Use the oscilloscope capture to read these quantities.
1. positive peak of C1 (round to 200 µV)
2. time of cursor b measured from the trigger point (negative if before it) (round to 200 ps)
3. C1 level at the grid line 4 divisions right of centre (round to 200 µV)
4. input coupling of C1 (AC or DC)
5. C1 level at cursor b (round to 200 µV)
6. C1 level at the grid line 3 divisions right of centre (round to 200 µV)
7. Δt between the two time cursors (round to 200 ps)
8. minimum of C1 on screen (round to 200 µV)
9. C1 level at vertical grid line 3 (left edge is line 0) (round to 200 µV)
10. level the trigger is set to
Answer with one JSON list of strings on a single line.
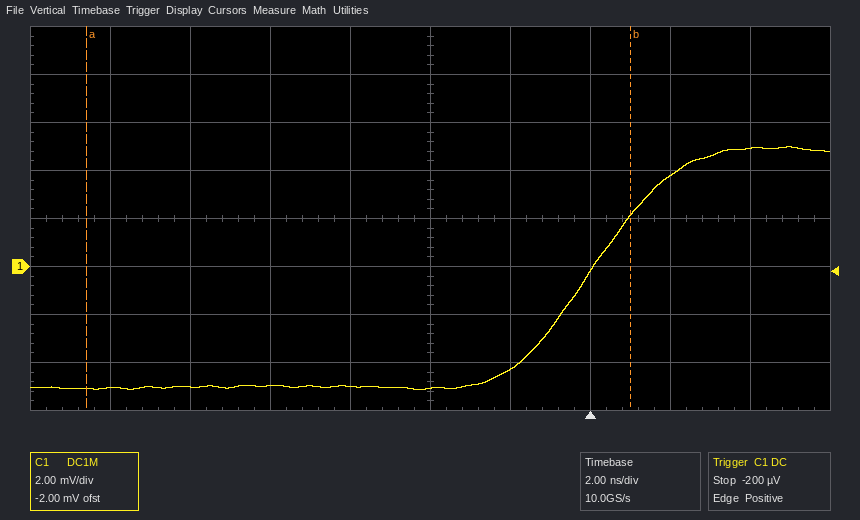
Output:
["5.0 mV", "+1.0 ns", "5.0 mV", "DC", "2.2 mV", "3.8 mV", "13.6 ns", "-5.2 mV", "-5.0 mV", "-200 µV"]
